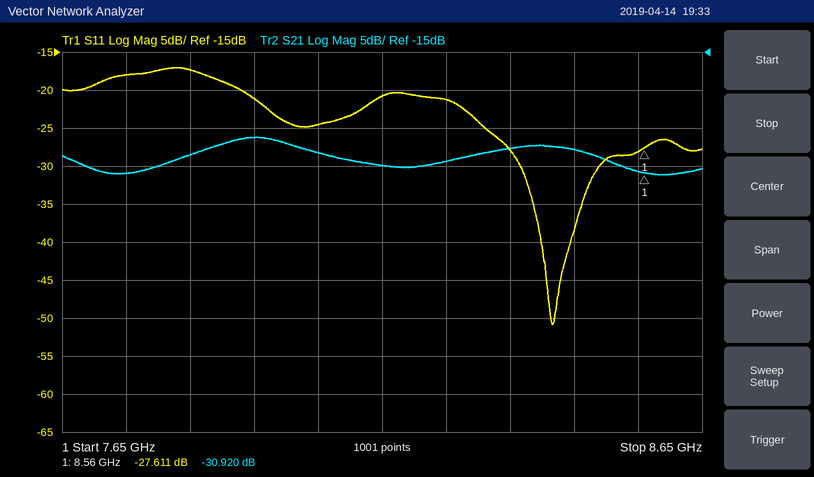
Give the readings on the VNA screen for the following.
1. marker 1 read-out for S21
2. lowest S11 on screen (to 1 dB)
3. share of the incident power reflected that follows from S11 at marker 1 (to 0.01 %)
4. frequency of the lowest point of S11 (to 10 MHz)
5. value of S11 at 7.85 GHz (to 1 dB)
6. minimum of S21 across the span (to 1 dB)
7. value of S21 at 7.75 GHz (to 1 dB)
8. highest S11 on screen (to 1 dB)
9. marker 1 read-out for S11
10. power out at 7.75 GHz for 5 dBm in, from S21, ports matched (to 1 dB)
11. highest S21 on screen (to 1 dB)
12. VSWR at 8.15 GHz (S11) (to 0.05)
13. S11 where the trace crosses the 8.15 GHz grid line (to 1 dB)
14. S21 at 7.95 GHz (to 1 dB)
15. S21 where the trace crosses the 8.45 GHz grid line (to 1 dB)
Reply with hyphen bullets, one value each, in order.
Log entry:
- -30.920 dB
- -51 dB
- 0.17 %
- 8.42 GHz
- -17 dB
- -31 dB
- -31 dB
- -17 dB
- -27.611 dB
- -26 dBm
- -26 dB
- 1.20
- -21 dB
- -26 dB
- -28 dB
